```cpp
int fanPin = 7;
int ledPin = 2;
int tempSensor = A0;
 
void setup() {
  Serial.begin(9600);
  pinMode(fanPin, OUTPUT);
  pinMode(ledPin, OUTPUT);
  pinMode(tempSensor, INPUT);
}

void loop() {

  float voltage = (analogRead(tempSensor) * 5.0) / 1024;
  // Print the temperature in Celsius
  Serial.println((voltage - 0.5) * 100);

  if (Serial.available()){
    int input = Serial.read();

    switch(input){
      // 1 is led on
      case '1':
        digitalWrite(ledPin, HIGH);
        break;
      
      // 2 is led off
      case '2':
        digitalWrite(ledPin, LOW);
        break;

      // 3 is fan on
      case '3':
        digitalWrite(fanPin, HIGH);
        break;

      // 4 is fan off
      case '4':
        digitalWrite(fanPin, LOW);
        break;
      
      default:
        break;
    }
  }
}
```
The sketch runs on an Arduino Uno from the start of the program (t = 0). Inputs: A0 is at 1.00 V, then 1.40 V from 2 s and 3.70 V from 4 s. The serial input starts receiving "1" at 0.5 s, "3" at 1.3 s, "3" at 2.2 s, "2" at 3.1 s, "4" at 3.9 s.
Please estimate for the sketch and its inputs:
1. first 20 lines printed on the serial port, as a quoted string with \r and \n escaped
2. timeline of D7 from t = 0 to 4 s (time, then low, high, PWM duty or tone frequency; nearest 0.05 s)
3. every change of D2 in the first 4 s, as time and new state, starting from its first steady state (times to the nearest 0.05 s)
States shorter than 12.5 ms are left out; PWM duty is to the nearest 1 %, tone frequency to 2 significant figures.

"49.61\r\n49.61\r\n49.61\r\n49.61\r\n49.61\r\n49.61\r\n49.61\r\n49.61\r\n49.61\r\n49.61\r\n49.61\r\n49.61\r\n49.61\r\n49.61\r\n49.61\r\n49.61\r\n49.61\r\n49.61\r\n49.61\r\n49.61\r\n"
0 s low; 1.3 s high; 3.9 s low
0 s low; 0.5 s high; 3.1 s low
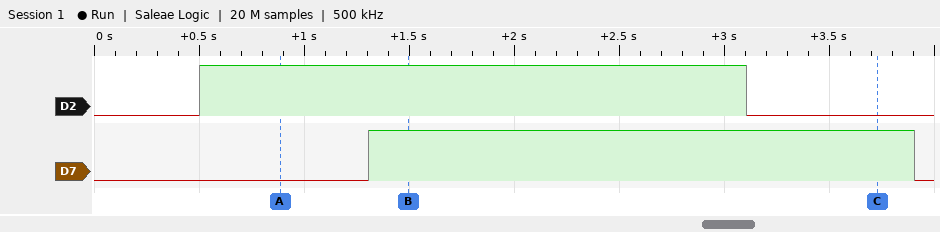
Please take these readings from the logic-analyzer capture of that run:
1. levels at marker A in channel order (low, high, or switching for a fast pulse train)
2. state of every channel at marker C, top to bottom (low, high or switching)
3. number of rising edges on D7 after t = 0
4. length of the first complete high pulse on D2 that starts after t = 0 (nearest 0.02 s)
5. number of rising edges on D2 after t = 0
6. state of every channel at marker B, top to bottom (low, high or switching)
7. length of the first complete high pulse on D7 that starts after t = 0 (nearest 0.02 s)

D2 high, D7 low
D2 low, D7 high
1
2.60 s
1
D2 high, D7 high
2.60 s
